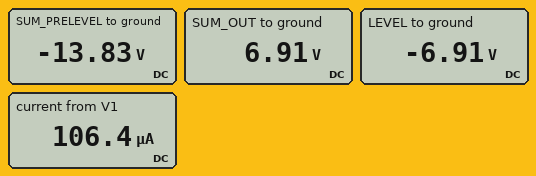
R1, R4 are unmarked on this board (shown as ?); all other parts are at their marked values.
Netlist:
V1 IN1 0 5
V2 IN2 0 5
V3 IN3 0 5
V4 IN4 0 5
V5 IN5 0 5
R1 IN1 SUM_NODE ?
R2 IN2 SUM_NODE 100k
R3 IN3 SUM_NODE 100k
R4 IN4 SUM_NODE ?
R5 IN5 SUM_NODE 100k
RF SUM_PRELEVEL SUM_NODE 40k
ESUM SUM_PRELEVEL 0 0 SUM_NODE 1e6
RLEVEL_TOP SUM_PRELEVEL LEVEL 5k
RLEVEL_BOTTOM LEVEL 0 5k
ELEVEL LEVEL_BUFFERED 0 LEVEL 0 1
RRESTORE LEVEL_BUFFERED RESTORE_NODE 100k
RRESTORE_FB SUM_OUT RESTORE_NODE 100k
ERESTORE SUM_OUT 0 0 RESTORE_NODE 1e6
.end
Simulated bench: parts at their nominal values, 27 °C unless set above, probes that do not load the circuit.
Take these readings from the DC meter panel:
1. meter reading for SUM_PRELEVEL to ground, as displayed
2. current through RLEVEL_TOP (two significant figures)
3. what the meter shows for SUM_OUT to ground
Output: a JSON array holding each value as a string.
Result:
["-13.83 V", "1.4 mA", "6.91 V"]
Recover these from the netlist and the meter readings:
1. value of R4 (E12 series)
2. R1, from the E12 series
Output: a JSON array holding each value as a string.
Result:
["56 kΩ", "47 kΩ"]
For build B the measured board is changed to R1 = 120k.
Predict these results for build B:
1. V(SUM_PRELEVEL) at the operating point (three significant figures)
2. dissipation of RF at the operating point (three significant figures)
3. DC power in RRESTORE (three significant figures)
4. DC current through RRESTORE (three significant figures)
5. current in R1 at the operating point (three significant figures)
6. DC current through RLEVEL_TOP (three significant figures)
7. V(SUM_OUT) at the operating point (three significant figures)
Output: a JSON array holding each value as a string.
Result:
["-11.2 V", "3.16 mW", "316 µW", "56.2 µA", "41.7 µA", "1.12 mA", "5.62 V"]
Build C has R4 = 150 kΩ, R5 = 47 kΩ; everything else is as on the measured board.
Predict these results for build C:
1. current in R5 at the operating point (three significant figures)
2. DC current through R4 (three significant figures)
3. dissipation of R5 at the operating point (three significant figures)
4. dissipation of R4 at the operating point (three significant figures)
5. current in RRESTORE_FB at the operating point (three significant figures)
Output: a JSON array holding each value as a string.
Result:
["106 µA", "33.3 µA", "532 µW", "167 µW", "69.2 µA"]
